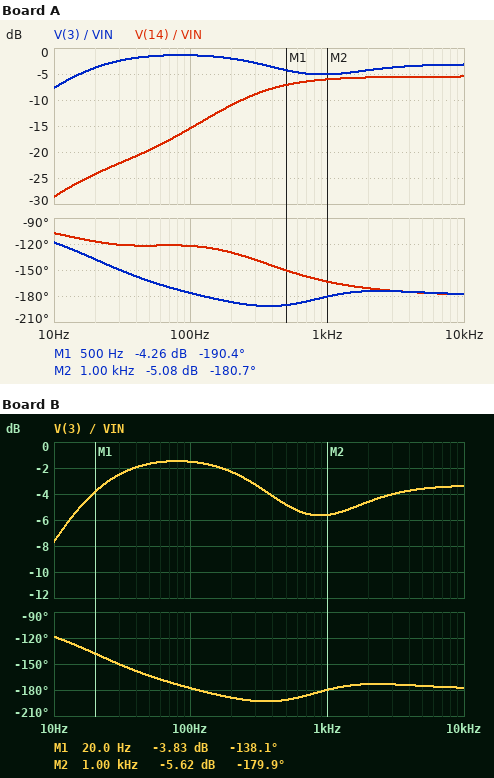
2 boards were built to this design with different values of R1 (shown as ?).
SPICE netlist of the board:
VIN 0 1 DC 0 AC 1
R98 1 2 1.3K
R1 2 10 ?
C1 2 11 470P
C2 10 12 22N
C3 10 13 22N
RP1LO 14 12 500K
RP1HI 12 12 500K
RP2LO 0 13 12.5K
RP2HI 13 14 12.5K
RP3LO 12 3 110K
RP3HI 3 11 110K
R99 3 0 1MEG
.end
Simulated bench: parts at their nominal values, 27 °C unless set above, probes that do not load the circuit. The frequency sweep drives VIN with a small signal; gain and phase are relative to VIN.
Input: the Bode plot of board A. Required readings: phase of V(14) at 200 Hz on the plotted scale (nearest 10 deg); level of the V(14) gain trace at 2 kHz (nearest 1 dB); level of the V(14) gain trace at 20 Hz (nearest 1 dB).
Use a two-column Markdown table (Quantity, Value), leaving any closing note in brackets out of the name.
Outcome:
| Quantity | Value |
|---|---|
| phase of V(14) at 200 Hz on the plotted scale | -130 deg |
| level of the V(14) gain trace at 2 kHz | -6 dB |
| level of the V(14) gain trace at 20 Hz | -24 dB |
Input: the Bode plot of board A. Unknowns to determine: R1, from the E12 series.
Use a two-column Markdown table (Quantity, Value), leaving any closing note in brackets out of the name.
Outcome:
| Quantity | Value |
|---|---|
| R1, from the E12 series | 10 kΩ |
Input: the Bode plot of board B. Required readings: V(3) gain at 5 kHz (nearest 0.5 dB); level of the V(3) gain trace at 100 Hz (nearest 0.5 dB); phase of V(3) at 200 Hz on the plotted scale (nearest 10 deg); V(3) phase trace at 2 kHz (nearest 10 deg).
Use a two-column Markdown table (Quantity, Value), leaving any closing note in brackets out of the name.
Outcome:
| Quantity | Value |
|---|---|
| V(3) gain at 5 kHz | -3.5 dB |
| level of the V(3) gain trace at 100 Hz | -1.5 dB |
| phase of V(3) at 200 Hz on the plotted scale | -190 deg |
| V(3) phase trace at 2 kHz | -170 deg |
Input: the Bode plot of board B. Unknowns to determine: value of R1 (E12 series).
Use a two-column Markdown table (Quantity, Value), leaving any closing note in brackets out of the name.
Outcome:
| Quantity | Value |
|---|---|
| value of R1 | 12 kΩ |
